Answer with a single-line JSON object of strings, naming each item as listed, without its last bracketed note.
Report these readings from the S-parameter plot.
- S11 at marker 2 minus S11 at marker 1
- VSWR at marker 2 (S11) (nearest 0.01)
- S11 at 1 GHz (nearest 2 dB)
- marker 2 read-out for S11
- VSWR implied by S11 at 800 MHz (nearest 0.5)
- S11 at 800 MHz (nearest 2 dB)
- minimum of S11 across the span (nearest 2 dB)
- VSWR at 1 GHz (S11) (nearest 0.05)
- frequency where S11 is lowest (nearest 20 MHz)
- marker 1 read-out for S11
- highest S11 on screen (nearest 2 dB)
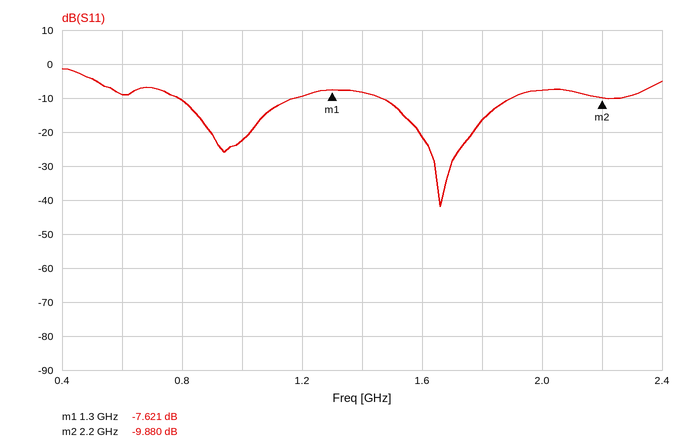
{"S11 at marker 2 minus S11 at marker 1": "-2.259 dB", "VSWR at marker 2 (S11)": "1.94", "S11 at 1 GHz": "-22 dB", "marker 2 read-out for S11": "-9.880 dB", "VSWR implied by S11 at 800 MHz": "2.0", "S11 at 800 MHz": "-10 dB", "minimum of S11 across the span": "-42 dB", "VSWR at 1 GHz (S11)": "1.15", "frequency where S11 is lowest": "1.66 GHz", "marker 1 read-out for S11": "-7.621 dB", "highest S11 on screen": "-2 dB"}
